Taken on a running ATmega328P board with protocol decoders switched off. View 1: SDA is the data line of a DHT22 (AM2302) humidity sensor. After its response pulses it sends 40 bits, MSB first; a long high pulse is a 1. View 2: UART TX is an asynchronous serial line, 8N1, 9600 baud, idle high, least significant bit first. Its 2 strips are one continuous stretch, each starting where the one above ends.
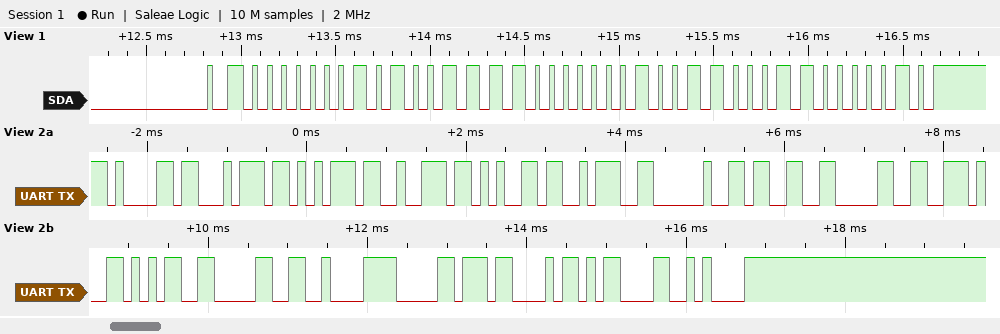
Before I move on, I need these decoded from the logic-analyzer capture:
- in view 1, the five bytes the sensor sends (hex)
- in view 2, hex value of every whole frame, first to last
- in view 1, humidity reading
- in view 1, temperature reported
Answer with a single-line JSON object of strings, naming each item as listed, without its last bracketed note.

{"in view 1, the five bytes the sensor sends": "01 4F 01 31 82", "in view 2, hex value of every whole frame, first to last": "61 74 75 72 65 3A 20 33 30 2E 35 30 C2 B0 43 0D 0A", "in view 1, humidity reading": "33.5 %", "in view 1, temperature reported": "30.5 °C"}
